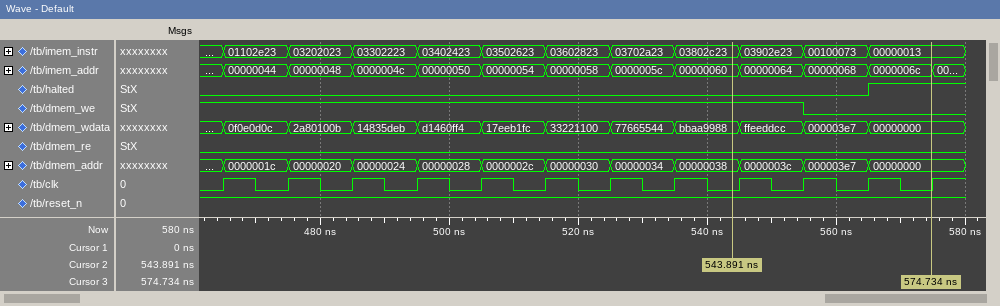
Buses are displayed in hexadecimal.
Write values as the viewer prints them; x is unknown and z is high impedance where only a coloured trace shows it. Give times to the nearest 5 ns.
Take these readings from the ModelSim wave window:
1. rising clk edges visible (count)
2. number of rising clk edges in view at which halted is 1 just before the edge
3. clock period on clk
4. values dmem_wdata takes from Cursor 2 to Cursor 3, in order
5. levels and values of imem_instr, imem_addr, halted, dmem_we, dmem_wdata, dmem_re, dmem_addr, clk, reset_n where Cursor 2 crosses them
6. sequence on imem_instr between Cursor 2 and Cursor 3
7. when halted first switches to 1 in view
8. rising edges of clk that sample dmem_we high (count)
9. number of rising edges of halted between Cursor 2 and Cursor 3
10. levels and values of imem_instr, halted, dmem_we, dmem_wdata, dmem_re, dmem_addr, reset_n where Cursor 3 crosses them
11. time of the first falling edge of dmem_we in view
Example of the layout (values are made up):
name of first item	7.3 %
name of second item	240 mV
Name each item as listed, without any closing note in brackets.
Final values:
rising clk edges visible	12
number of rising clk edges in view at which halted is 1 just before the edge	1
clock period on clk	10 ns
values dmem_wdata takes from Cursor 2 to Cursor 3, in order	bbaa9988, ffeeddcc, 000003e7, 00000000
levels and values of imem_instr, imem_addr, halted, dmem_we, dmem_wdata, dmem_re, dmem_addr, clk, reset_n where Cursor 2 crosses them	imem_instr=03802c23, imem_addr=00000060, halted=0, dmem_we=1, dmem_wdata=bbaa9988, dmem_re=0, dmem_addr=00000038, clk=0, reset_n=1
sequence on imem_instr between Cursor 2 and Cursor 3	03802c23, 03902e23, 00100073, 00000013
when halted first switches to 1 in view	565 ns
rising edges of clk that sample dmem_we high	10
number of rising edges of halted between Cursor 2 and Cursor 3	1
levels and values of imem_instr, halted, dmem_we, dmem_wdata, dmem_re, dmem_addr, reset_n where Cursor 3 crosses them	imem_instr=00000013, halted=1, dmem_we=0, dmem_wdata=00000000, dmem_re=0, dmem_addr=00000000, reset_n=1
time of the first falling edge of dmem_we in view	555 ns
